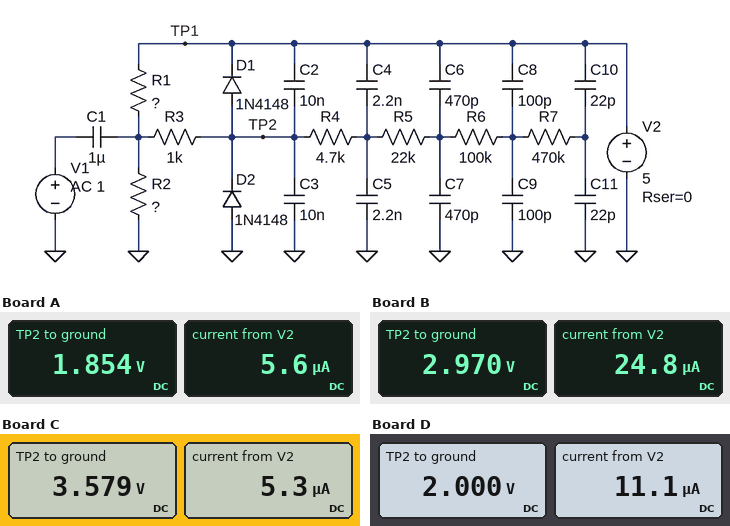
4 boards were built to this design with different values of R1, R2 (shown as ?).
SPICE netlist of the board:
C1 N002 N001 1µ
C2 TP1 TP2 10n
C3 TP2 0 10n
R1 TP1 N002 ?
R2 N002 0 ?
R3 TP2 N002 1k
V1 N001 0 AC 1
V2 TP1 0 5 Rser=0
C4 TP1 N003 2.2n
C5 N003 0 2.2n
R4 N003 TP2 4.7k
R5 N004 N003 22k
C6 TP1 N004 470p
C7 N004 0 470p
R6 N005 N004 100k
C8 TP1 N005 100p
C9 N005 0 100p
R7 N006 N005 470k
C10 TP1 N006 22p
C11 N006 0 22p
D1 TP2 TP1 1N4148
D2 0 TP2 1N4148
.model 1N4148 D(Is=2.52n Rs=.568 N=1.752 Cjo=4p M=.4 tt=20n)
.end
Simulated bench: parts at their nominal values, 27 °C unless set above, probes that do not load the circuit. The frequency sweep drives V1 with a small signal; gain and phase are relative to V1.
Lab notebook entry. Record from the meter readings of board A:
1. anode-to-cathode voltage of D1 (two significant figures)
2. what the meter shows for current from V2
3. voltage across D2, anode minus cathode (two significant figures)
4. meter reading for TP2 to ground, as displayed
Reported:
-3.1 V
5.6 µA
-1.9 V
1.854 V
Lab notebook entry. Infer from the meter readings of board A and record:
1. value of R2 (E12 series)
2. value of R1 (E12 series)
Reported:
330 kΩ
560 kΩ
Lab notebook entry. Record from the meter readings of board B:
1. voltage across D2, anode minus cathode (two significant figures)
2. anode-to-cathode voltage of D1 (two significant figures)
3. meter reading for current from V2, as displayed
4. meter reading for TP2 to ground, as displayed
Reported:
-3.0 V
-2.0 V
24.8 µA
2.970 V
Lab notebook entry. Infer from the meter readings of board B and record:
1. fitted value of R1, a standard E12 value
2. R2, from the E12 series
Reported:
82 kΩ
120 kΩ
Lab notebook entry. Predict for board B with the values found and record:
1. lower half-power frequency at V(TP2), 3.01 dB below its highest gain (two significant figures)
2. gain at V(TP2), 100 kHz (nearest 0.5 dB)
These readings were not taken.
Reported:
3.2 Hz
-22.0 dB
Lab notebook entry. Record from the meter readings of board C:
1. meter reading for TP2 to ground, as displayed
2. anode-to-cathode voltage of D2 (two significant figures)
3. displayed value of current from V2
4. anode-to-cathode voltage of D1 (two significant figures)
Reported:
3.579 V
-3.6 V
5.3 µA
-1.4 V
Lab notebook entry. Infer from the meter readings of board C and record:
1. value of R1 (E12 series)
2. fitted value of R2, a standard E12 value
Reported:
270 kΩ
680 kΩ
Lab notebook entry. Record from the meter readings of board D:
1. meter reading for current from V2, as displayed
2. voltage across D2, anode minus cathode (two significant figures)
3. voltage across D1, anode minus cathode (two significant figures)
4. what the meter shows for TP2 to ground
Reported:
11.1 µA
-2.0 V
-3.0 V
2.000 V
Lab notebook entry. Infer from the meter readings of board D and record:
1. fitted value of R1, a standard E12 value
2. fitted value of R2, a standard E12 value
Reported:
270 kΩ
180 kΩ
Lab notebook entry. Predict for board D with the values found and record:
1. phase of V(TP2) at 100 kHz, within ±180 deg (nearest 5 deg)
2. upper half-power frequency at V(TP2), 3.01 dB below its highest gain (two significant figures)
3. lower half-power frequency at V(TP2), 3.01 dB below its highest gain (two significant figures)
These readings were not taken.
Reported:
-85 deg
6.6 kHz
1.4 Hz
